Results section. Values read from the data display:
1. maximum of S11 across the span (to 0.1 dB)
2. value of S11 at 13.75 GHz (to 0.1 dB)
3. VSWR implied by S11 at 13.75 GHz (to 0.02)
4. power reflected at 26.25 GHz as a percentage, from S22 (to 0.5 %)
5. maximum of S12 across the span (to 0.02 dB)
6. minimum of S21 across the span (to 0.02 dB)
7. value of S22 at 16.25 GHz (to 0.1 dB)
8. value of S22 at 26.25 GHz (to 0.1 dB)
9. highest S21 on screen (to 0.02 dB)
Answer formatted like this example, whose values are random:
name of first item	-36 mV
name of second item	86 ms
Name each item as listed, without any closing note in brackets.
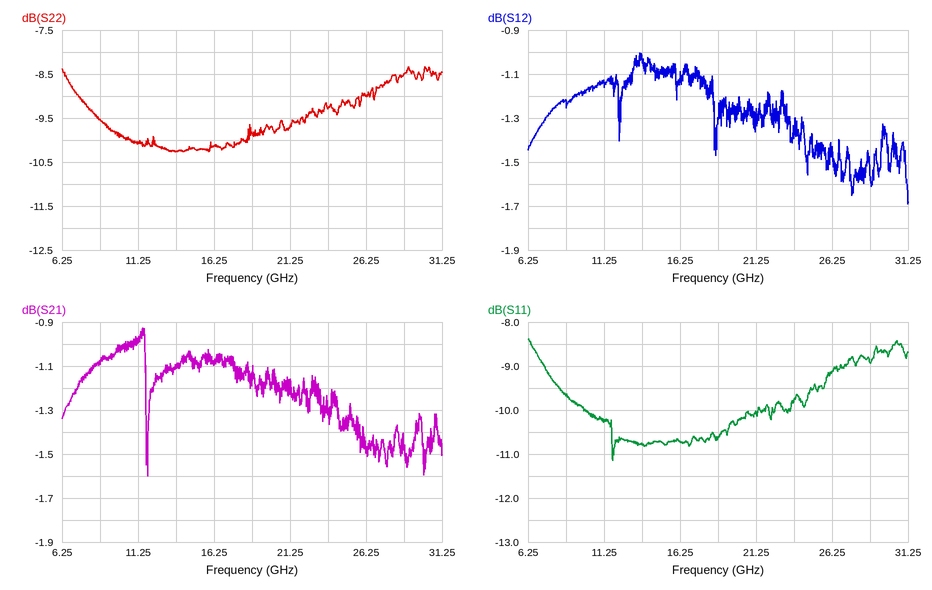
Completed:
maximum of S11 across the span	-8.4 dB
value of S11 at 13.75 GHz	-10.8 dB
VSWR implied by S11 at 13.75 GHz	1.82
power reflected at 26.25 GHz as a percentage, from S22	12.5 %
maximum of S12 across the span	-1.00 dB
minimum of S21 across the span	-1.60 dB
value of S22 at 16.25 GHz	-10.1 dB
value of S22 at 26.25 GHz	-9.0 dB
highest S21 on screen	-0.92 dB
